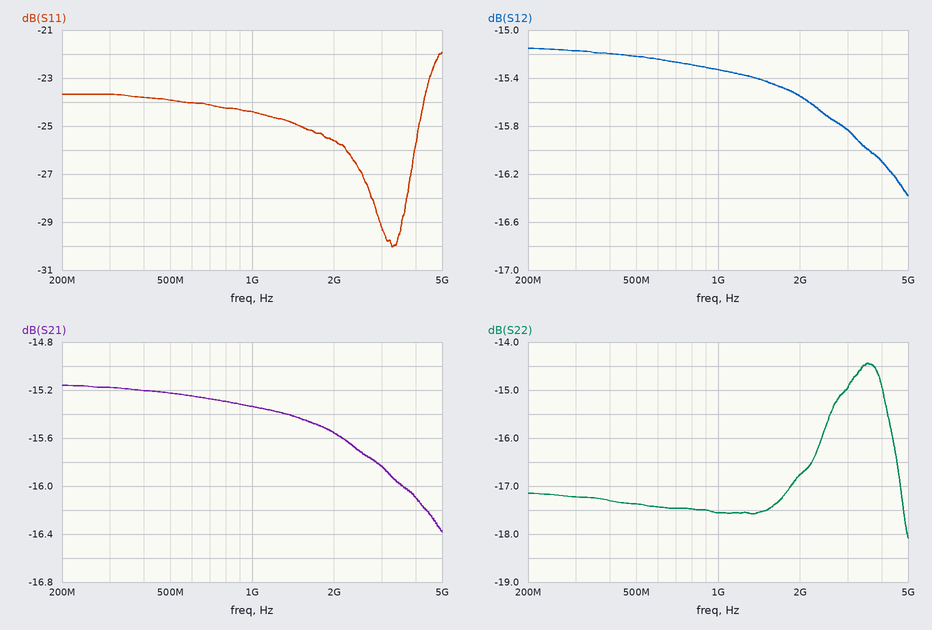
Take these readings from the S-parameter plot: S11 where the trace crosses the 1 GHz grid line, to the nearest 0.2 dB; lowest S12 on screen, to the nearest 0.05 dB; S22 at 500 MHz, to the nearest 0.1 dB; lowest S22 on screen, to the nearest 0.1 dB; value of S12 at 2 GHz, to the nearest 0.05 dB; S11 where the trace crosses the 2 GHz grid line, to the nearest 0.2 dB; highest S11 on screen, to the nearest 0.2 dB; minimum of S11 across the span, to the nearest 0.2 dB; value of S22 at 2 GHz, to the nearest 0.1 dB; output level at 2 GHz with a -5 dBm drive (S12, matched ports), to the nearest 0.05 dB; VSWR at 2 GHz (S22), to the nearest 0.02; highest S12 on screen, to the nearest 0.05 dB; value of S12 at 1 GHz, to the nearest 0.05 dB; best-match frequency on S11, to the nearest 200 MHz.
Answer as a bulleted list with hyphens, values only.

- -24.4 dB
- -16.40 dB
- -17.4 dB
- -18.1 dB
- -15.55 dB
- -25.6 dB
- -22.0 dB
- -30.0 dB
- -16.8 dB
- -20.55 dBm
- 1.34
- -15.15 dB
- -15.35 dB
- 3.2 GHz
